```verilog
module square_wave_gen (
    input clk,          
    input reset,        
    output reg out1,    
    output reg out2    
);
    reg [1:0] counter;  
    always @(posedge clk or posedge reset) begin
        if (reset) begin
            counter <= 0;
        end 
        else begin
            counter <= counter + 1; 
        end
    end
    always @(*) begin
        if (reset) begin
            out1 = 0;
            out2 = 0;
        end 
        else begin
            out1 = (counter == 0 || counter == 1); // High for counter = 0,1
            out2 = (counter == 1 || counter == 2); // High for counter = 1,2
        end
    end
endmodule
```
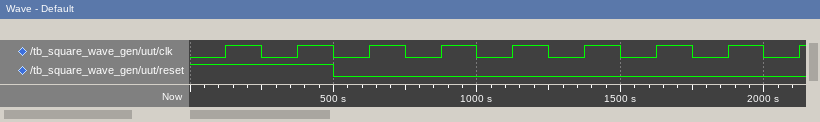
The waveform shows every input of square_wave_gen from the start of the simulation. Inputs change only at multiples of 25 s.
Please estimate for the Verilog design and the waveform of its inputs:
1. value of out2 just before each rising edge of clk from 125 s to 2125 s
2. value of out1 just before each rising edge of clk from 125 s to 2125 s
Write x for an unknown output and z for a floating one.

0 0 0 1 1 0 0 1 1
0 0 1 1 0 0 1 1 0
